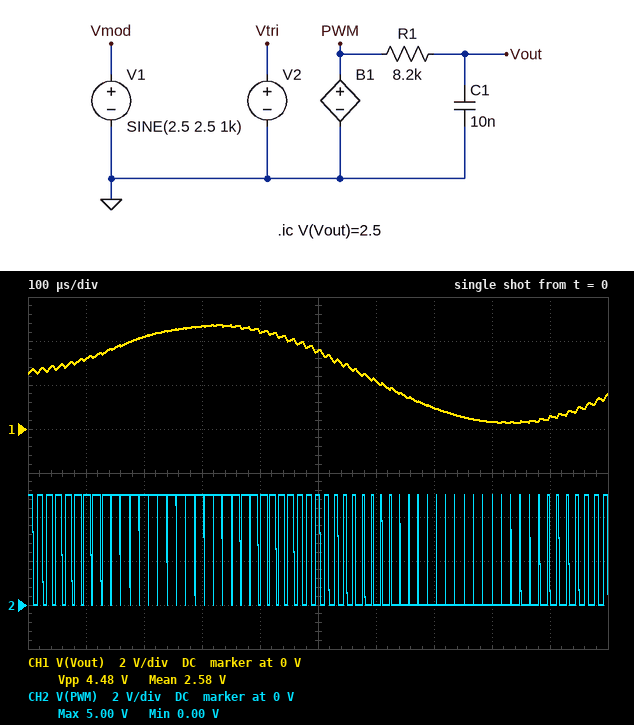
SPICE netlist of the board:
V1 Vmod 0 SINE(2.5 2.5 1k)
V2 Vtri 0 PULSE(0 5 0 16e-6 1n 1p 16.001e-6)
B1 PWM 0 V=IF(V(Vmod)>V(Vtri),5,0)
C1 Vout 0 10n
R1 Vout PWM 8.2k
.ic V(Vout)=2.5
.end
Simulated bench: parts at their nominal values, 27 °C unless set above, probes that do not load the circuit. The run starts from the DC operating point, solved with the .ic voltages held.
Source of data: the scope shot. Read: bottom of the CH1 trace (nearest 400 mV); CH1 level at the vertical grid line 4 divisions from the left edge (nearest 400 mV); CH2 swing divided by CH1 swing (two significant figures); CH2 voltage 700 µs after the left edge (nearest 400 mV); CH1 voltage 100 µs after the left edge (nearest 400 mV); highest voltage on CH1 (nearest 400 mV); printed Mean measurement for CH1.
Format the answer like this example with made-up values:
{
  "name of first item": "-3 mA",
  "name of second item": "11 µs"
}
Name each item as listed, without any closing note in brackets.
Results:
{
  "bottom of the CH1 trace": "400 mV",
  "CH1 level at the vertical grid line 4 divisions from the left edge": "4.4 V",
  "CH2 swing divided by CH1 swing": "1.1",
  "CH2 voltage 700 µs after the left edge": "0 V",
  "CH1 voltage 100 µs after the left edge": "3.2 V",
  "highest voltage on CH1": "4.8 V",
  "printed Mean measurement for CH1": "2.58 V"
}
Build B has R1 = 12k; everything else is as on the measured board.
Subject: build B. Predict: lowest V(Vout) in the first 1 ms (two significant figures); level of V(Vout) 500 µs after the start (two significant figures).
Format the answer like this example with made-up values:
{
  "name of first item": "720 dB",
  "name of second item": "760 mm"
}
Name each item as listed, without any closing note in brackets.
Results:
{
  "lowest V(Vout) in the first 1 ms": "480 mV",
  "level of V(Vout) 500 µs after the start": "3.7 V"
}
